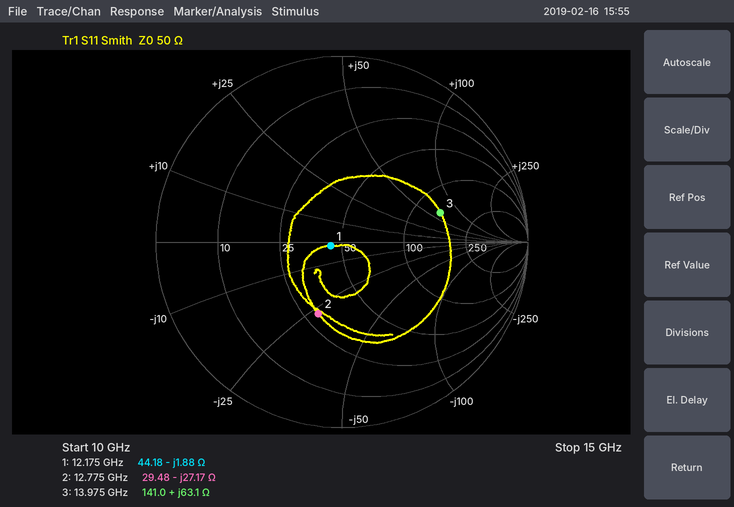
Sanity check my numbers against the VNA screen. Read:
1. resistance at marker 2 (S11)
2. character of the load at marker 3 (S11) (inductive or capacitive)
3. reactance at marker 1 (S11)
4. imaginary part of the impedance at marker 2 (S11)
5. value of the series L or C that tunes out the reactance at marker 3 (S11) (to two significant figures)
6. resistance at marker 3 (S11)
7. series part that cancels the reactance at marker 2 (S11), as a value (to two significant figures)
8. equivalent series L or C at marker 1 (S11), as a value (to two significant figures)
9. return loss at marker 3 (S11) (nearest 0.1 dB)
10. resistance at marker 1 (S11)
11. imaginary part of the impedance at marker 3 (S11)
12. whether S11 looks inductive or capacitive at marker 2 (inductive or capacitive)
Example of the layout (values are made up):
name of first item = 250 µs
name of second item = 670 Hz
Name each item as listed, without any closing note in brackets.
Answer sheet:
resistance at marker 2 = 29.48 Ω
character of the load at marker 3 (S11) = inductive
reactance at marker 1 = -1.88 Ω
imaginary part of the impedance at marker 2 = -27.17 Ω
value of the series L or C that tunes out the reactance at marker 3 (S11) = 180 fF
resistance at marker 3 = 141.0 Ω
series part that cancels the reactance at marker 2 (S11), as a value = 340 pH
equivalent series L or C at marker 1 (S11), as a value = 7.0 pF
return loss at marker 3 (S11) = 5.2 dB
resistance at marker 1 = 44.18 Ω
imaginary part of the impedance at marker 3 = +63.1 Ω
whether S11 looks inductive or capacitive at marker 2 = capacitive
